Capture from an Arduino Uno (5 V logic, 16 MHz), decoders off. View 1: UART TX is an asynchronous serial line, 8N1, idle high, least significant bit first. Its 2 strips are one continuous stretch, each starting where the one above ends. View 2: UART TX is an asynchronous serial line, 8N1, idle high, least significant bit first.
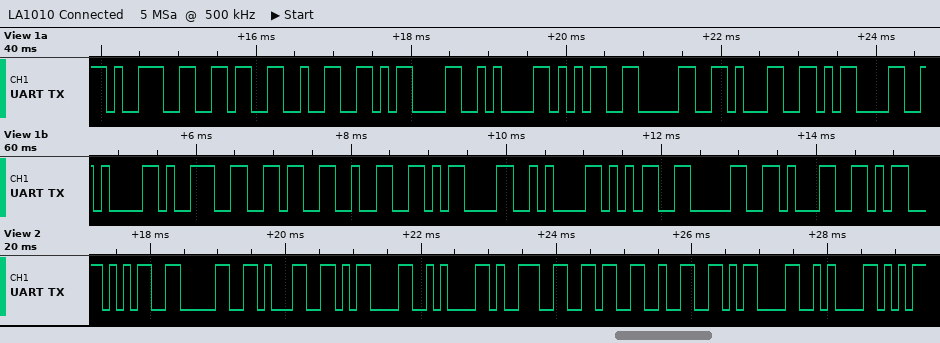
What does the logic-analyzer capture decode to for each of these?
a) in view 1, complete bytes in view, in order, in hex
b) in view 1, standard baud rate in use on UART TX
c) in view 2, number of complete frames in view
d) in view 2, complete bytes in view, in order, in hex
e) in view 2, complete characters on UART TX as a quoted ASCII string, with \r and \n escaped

39 36 32 0D 0A 35 30 31 0D 0A 39 36 32 0D 0A 35 30 31
9600 baud
10
0x35 0x30 0x31 0x0D 0x0A 0x39 0x36 0x32 0x0D 0x0A
"501\r\n962\r\n"
